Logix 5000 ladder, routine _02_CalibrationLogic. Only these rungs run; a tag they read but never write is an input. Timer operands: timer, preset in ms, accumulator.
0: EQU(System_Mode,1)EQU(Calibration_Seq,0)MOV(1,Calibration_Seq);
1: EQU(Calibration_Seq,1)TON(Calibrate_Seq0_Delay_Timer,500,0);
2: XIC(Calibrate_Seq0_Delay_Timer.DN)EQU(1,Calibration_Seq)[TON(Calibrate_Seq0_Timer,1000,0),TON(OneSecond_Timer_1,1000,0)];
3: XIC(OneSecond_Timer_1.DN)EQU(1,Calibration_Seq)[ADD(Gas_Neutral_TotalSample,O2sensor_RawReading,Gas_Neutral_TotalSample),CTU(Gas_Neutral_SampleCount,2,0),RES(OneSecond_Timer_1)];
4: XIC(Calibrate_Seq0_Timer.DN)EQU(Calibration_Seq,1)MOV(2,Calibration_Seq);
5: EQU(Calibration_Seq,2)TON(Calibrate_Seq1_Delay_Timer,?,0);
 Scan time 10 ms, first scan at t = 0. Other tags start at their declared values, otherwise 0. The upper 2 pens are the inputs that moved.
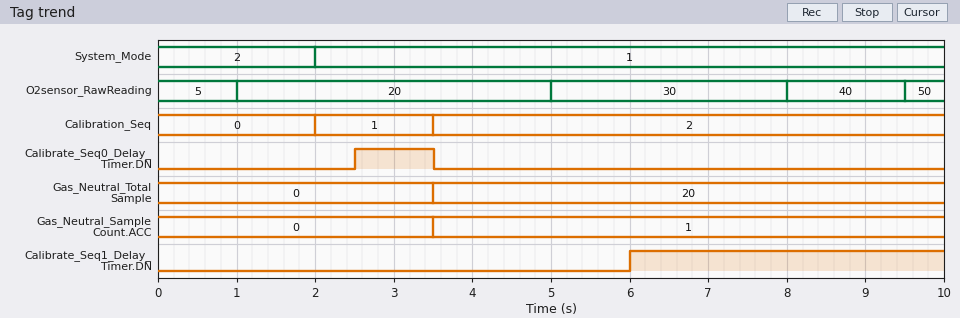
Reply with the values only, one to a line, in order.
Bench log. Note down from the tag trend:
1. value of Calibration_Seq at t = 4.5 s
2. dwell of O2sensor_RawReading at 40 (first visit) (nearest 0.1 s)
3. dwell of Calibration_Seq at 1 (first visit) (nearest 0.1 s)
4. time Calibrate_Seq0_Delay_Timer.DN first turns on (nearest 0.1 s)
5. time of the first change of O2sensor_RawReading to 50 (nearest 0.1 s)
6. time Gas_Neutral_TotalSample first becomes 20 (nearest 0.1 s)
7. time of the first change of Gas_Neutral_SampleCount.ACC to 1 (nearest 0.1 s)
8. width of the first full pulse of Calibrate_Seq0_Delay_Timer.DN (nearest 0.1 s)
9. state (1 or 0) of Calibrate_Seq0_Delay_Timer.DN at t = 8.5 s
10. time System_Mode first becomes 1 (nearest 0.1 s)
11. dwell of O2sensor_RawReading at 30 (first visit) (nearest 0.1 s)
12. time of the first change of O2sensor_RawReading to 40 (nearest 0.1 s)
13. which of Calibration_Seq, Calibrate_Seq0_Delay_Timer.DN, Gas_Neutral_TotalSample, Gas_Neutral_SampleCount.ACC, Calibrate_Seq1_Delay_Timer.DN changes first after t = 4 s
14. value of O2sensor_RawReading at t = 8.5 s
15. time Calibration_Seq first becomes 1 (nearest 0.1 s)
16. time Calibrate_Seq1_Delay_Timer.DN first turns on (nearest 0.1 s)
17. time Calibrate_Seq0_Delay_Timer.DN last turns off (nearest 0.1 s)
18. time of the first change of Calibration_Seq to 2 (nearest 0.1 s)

2
1.5 s
1.5 s
2.5 s
9.5 s
3.5 s
3.5 s
1.0 s
0
2.0 s
3.0 s
8.0 s
Calibrate_Seq1_Delay_Timer.DN
40
2.0 s
6.0 s
3.5 s
3.5 s
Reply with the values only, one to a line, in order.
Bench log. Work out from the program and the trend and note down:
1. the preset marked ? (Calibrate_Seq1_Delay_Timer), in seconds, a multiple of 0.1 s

2.5 s
